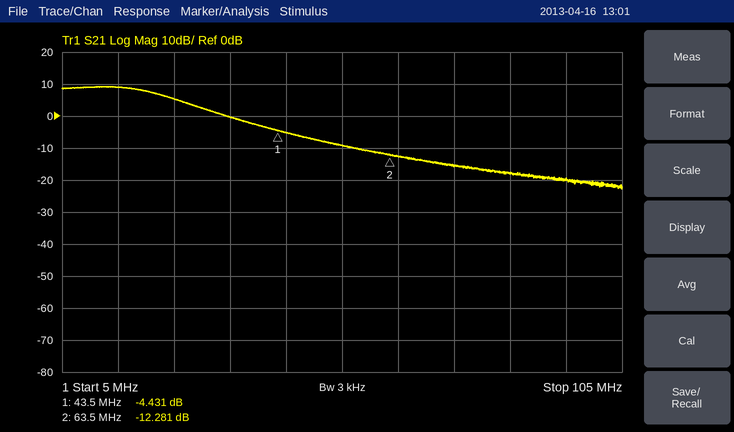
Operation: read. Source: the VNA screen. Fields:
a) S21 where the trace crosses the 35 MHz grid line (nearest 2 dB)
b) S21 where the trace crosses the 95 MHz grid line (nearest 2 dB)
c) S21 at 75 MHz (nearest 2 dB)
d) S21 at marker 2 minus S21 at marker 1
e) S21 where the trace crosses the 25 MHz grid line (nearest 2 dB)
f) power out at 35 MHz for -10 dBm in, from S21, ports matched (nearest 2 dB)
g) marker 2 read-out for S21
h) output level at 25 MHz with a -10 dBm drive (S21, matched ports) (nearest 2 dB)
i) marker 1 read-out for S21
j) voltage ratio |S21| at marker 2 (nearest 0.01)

0 dB
-20 dB
-16 dB
-7.850 dB
6 dB
-10 dBm
-12.281 dB
-4 dBm
-4.431 dB
0.24
